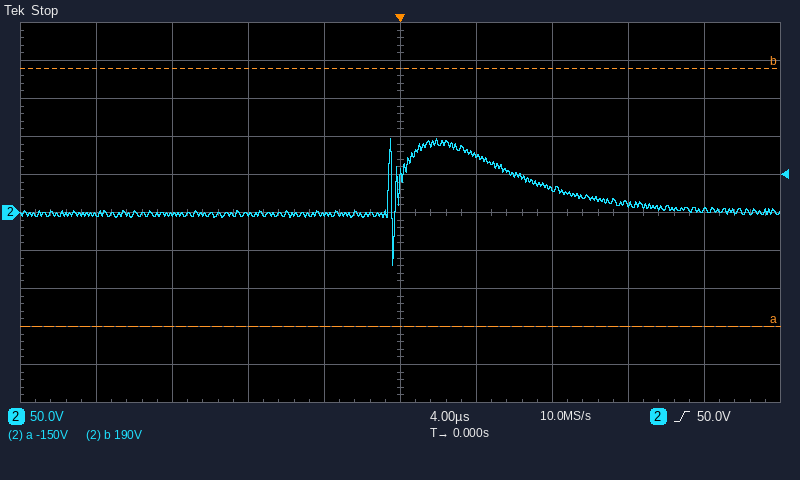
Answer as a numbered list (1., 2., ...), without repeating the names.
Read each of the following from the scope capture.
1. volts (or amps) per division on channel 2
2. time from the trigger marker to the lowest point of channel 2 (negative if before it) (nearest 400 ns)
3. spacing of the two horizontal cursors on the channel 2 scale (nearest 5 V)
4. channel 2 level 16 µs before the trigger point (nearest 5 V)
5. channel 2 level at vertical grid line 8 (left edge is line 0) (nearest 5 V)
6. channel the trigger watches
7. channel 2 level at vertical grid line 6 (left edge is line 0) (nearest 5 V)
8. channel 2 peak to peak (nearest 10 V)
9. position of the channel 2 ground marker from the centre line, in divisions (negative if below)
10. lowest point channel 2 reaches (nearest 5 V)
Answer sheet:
1. 50 V
2. -400 ns
3. 340 V
4. 0 V
5. 10 V
6. channel 2
7. 75 V
8. 170 V
9. 0.0 div
10. -70 V
